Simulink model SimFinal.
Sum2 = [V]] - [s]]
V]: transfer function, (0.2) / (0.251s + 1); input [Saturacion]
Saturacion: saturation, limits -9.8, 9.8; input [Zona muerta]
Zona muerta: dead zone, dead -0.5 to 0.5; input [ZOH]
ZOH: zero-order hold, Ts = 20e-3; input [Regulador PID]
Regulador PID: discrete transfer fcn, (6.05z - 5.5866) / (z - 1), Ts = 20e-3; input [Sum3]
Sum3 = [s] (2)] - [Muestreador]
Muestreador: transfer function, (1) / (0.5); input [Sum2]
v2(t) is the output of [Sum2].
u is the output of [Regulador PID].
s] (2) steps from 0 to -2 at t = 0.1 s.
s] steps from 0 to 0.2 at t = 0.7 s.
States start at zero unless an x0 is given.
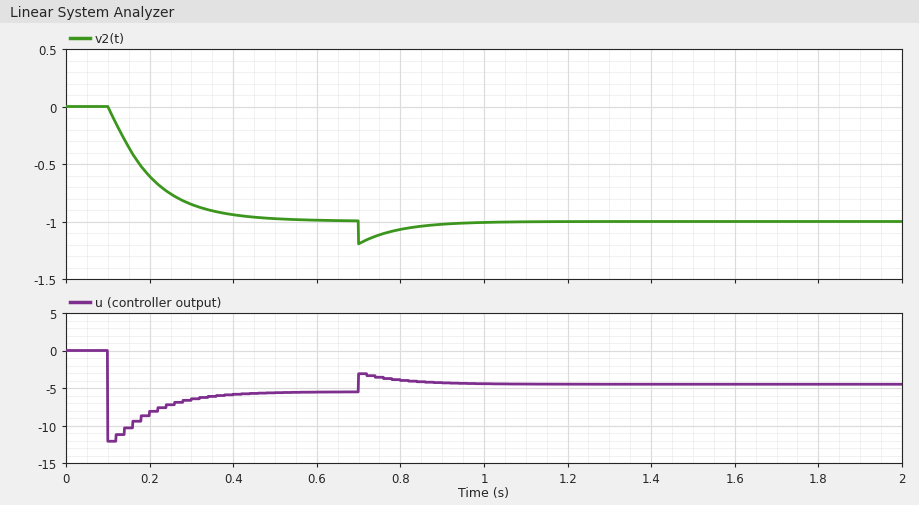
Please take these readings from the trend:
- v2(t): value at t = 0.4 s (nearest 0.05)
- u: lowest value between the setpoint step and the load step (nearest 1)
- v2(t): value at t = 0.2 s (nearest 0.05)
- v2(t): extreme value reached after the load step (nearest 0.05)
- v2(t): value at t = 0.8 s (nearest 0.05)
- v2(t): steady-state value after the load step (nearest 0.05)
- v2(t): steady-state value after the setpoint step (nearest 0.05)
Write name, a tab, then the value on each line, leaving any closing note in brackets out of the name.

v2(t): value at t = 0.4 s	-0.95
u: lowest value between the setpoint step and the load step	-12
v2(t): value at t = 0.2 s	-0.60
v2(t): extreme value reached after the load step	-1.20
v2(t): value at t = 0.8 s	-1.05
v2(t): steady-state value after the load step	-1.00
v2(t): steady-state value after the setpoint step	-1.00
